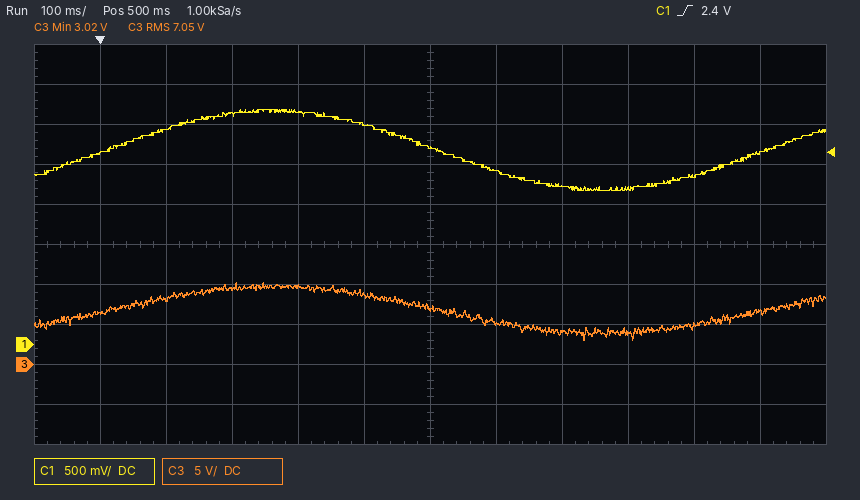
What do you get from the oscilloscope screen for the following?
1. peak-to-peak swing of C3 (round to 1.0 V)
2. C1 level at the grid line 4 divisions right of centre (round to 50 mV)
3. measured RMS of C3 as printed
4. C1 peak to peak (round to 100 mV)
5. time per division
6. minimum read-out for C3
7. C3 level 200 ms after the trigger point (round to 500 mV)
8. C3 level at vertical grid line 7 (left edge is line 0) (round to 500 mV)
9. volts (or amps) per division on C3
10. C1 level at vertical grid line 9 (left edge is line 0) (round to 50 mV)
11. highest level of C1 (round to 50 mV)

7.0 V
2.10 V
7.05 V
1.00 V
100 ms
3.02 V
9.5 V
5.0 V
5 V
1.95 V
2.95 V
